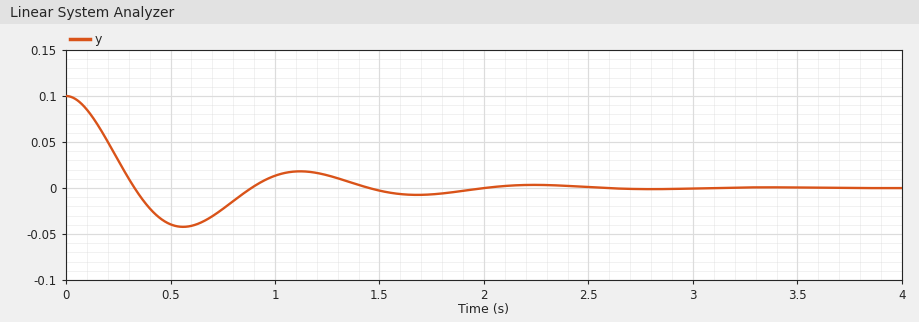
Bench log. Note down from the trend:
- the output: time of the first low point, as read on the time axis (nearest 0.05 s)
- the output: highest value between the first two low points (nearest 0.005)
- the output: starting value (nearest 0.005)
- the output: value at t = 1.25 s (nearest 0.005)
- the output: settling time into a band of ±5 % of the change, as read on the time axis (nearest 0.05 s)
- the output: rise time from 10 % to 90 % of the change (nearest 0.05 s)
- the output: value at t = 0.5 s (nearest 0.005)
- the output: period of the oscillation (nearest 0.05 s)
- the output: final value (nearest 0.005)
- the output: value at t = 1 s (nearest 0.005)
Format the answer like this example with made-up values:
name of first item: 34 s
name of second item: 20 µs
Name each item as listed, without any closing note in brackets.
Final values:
the output: time of the first low point, as read on the time axis: 0.55 s
the output: highest value between the first two low points: 0.020
the output: starting value: 0.100
the output: value at t = 1.25 s: 0.015
the output: settling time into a band of ±5 % of the change, as read on the time axis: 1.85 s
the output: rise time from 10 % to 90 % of the change: 0.20 s
the output: value at t = 0.5 s: -0.040
the output: period of the oscillation: 1.10 s
the output: final value: 0.000
the output: value at t = 1 s: 0.015
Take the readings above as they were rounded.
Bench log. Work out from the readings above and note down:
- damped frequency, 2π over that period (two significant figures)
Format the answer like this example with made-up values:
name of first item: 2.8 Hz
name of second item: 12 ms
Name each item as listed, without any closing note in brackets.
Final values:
damped frequency, 2π over that period: 5.7 rad/s
